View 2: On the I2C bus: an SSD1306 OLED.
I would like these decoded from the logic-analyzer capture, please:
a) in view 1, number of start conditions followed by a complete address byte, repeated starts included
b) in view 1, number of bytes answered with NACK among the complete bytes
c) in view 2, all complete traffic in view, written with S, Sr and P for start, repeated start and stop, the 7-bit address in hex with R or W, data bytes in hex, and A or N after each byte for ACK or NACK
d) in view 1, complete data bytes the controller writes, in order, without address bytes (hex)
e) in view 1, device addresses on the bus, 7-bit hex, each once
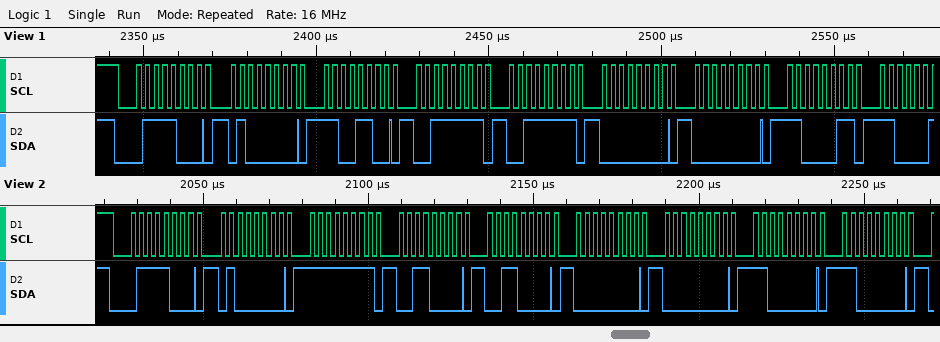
1
0
S 3CW A 40 A FF A 30 A 30 A 00 A 00 A C0 A C0 A
40 CC 3F 3F 00 00 C3
0x3C
